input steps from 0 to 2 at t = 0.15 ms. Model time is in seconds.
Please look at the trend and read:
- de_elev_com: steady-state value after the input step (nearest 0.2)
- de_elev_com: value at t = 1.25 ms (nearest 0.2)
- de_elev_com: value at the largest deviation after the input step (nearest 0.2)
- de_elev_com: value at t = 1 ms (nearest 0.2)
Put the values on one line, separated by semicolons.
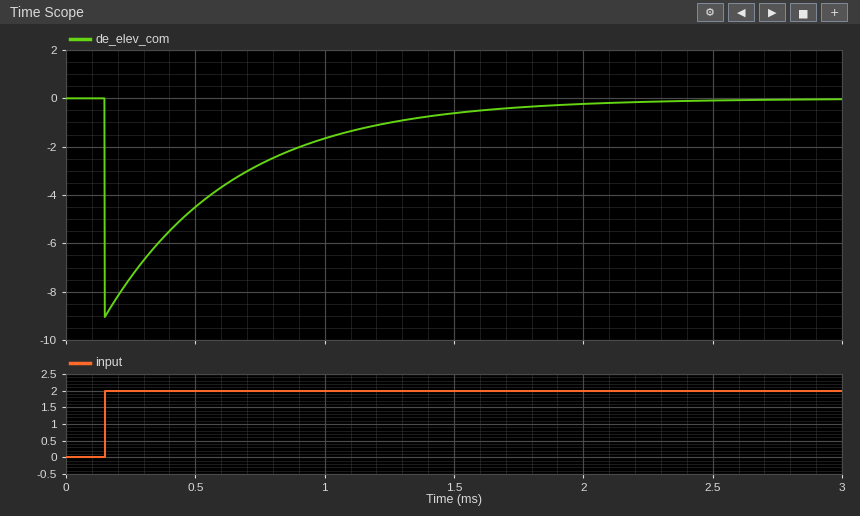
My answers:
0.0; -1.0; -9.0; -1.6
